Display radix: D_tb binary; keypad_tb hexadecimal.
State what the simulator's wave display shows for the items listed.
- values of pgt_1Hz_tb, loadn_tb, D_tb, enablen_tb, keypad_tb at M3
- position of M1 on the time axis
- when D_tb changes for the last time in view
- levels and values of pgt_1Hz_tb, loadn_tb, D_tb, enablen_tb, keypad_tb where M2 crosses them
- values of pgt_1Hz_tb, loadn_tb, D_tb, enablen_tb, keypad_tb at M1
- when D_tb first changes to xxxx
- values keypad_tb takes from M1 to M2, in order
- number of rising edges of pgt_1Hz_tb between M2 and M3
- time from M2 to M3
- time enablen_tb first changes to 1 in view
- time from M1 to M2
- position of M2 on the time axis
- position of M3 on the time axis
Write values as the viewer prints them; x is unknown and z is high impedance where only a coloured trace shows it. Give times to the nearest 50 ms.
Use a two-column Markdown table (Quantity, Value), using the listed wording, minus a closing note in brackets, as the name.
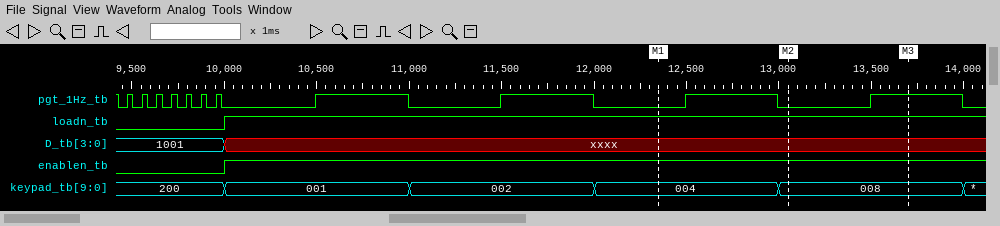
| Quantity | Value |
|---|---|
| values of pgt_1Hz_tb, loadn_tb, D_tb, enablen_tb, keypad_tb at M3 | pgt_1Hz_tb=1, loadn_tb=1, D_tb=xxxx, enablen_tb=1, keypad_tb=008 |
| position of M1 on the time axis | 12350 ms |
| when D_tb changes for the last time in view | 10000 ms |
| levels and values of pgt_1Hz_tb, loadn_tb, D_tb, enablen_tb, keypad_tb where M2 crosses them | pgt_1Hz_tb=0, loadn_tb=1, D_tb=xxxx, enablen_tb=1, keypad_tb=008 |
| values of pgt_1Hz_tb, loadn_tb, D_tb, enablen_tb, keypad_tb at M1 | pgt_1Hz_tb=0, loadn_tb=1, D_tb=xxxx, enablen_tb=1, keypad_tb=004 |
| when D_tb first changes to xxxx | 10000 ms |
| values keypad_tb takes from M1 to M2, in order | 004, 008 |
| number of rising edges of pgt_1Hz_tb between M2 and M3 | 1 |
| time from M2 to M3 | 650 ms |
| time enablen_tb first changes to 1 in view | 10000 ms |
| time from M1 to M2 | 700 ms |
| position of M2 on the time axis | 13050 ms |
| position of M3 on the time axis | 13700 ms |
